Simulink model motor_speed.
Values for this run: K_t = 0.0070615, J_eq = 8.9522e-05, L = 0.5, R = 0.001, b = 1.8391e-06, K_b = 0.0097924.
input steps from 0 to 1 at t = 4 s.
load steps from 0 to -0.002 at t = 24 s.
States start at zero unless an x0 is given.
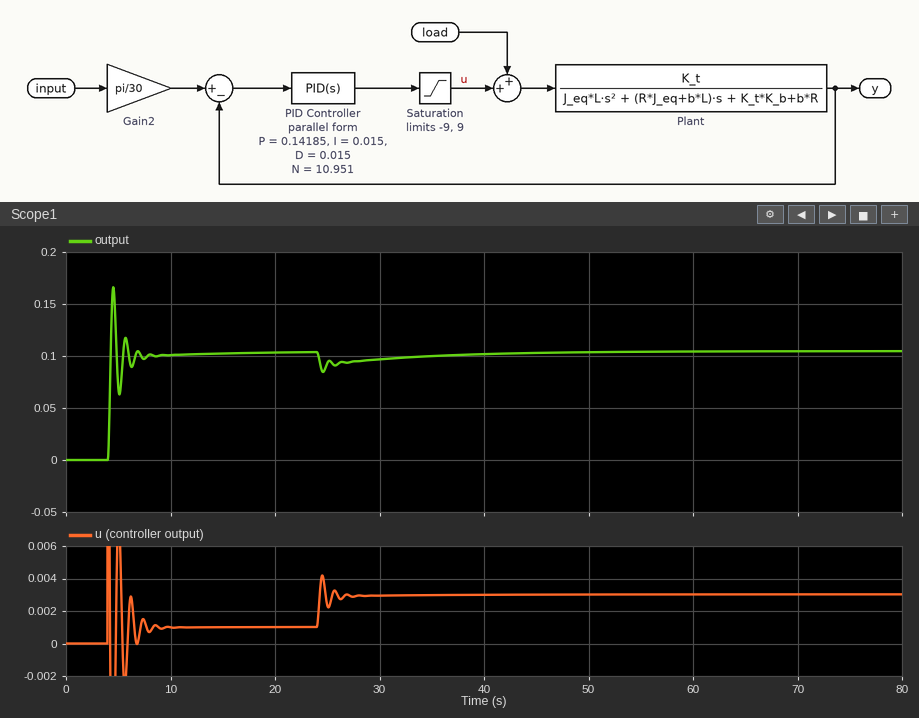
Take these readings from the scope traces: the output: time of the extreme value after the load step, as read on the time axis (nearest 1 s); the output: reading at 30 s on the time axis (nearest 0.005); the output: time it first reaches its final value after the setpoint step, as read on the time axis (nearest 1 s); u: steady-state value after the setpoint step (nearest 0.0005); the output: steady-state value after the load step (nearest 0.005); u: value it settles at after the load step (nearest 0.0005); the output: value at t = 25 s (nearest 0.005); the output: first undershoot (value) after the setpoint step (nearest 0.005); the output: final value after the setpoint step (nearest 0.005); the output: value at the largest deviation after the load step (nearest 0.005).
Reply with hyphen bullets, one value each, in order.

- 25 s
- 0.095
- 4 s
- 0.0010
- 0.105
- 0.0030
- 0.095
- 0.065
- 0.105
- 0.085
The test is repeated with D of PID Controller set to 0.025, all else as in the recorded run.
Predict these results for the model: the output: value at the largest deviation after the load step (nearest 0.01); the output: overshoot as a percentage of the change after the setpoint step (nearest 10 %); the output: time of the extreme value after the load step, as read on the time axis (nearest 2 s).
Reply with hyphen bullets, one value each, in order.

- 0.09
- 50 %
- 24 s
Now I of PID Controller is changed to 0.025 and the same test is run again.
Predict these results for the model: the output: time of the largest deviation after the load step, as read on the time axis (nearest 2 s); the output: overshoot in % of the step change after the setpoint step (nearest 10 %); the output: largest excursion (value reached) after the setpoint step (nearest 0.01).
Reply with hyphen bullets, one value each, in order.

- 24 s
- 60 %
- 0.17
